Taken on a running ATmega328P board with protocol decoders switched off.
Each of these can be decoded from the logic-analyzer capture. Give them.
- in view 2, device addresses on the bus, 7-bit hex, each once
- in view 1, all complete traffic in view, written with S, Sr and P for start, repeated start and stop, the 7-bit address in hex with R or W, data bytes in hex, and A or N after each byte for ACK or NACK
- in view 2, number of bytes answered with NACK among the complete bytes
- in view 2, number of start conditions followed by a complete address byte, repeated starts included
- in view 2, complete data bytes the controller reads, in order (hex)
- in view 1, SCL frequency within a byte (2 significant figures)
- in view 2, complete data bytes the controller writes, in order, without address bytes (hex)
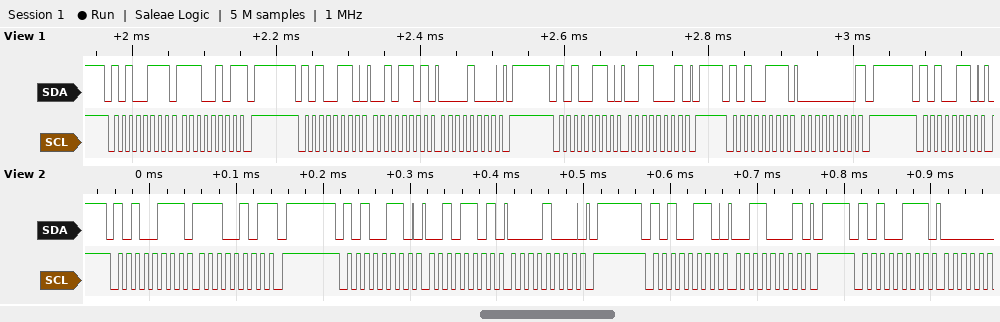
0x53
S 53R A E5 N P S 53W A 2D A 08 A P S 53W A 31 A P S 53R A 00 N P S 53W A
1
4
E5
100 kHz
2D 08 31
